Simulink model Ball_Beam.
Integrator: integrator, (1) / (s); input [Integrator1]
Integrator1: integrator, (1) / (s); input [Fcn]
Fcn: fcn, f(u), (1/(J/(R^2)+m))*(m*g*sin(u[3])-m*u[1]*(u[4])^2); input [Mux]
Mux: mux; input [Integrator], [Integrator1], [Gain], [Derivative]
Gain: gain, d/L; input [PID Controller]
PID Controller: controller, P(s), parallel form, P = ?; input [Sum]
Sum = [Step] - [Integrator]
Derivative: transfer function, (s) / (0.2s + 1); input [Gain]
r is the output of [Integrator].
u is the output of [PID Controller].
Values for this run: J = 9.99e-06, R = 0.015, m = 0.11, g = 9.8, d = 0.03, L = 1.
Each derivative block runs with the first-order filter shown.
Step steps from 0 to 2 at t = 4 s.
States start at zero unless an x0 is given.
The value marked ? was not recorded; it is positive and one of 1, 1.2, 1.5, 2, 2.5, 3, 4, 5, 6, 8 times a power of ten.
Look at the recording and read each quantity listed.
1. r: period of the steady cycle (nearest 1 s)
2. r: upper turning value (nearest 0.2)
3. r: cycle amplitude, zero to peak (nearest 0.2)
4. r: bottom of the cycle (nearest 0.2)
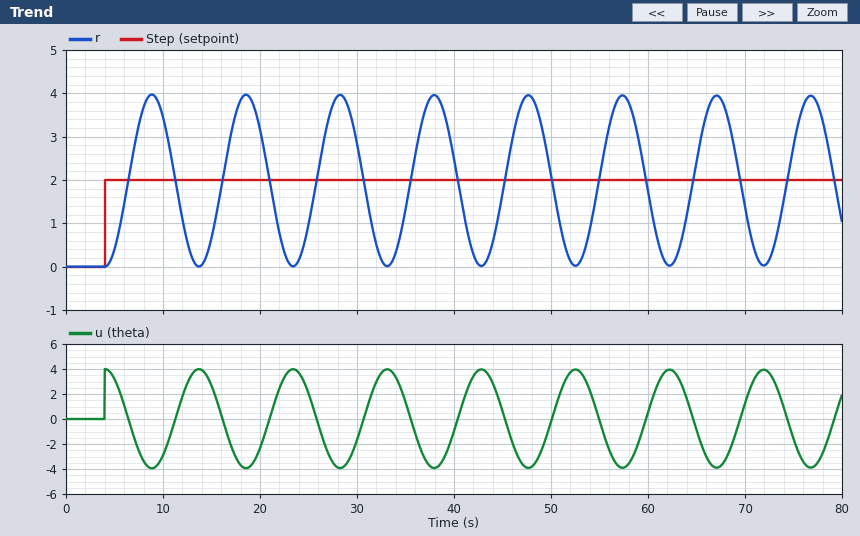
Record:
10 s
4.0
2.0
0.0
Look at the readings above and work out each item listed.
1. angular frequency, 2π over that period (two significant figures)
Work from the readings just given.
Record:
0.63 rad/s
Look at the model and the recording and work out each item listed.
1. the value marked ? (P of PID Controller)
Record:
2
